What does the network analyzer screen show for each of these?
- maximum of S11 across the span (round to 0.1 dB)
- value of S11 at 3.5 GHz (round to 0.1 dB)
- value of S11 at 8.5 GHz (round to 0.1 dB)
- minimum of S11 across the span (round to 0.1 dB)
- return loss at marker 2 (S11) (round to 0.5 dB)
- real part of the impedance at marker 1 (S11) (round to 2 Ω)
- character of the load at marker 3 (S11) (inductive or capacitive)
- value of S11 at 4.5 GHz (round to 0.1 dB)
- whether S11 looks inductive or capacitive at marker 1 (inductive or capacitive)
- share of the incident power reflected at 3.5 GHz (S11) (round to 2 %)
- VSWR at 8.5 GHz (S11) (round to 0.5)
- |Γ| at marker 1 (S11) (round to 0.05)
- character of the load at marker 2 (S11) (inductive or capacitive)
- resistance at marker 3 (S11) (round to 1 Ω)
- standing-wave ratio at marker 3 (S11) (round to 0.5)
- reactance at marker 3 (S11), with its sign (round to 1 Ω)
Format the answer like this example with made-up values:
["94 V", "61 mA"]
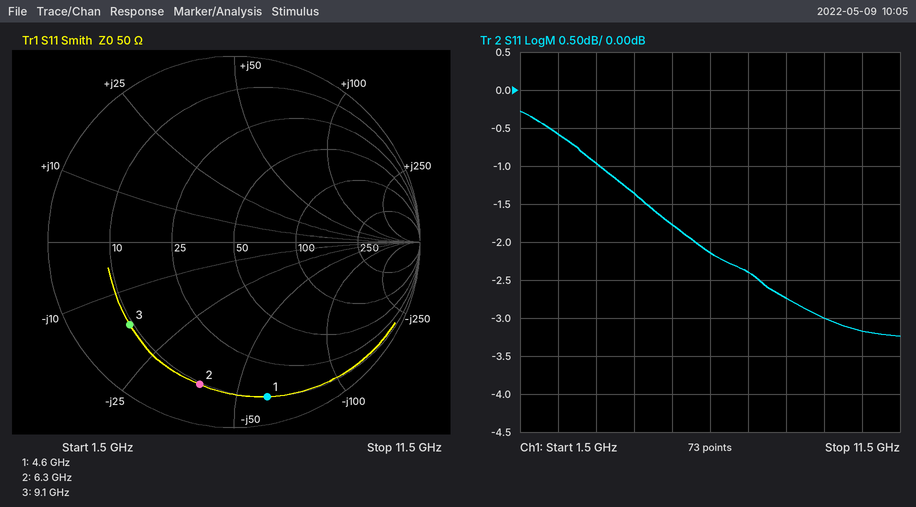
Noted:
["-0.3 dB", "-1.0 dB", "-2.7 dB", "-3.2 dB", "2.0 dB", "10 Ω", "capacitive", "-1.4 dB", "capacitive", "80 %", "6.5", "0.85", "capacitive", "9 Ω", "6.0", "-17 Ω"]
